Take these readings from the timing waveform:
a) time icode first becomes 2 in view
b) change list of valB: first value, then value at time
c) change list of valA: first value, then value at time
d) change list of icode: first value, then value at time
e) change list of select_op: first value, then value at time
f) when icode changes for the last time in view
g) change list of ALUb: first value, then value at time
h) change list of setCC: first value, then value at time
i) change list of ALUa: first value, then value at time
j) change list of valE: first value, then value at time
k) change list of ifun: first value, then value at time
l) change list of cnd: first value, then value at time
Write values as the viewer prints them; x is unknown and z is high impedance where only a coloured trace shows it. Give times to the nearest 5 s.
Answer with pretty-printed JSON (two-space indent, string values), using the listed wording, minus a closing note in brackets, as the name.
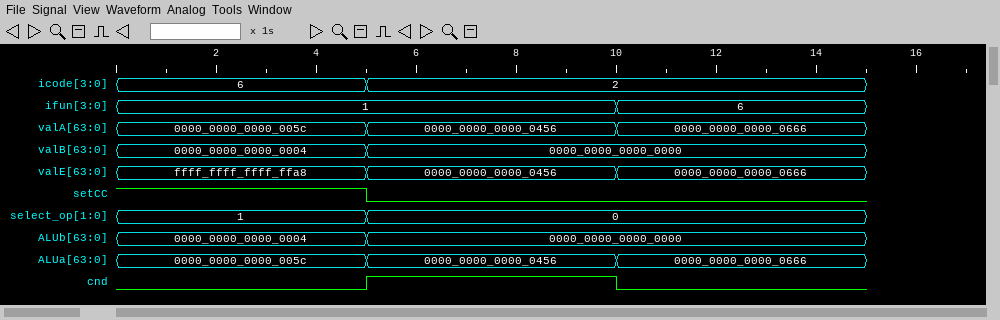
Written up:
{
  "time icode first becomes 2 in view": "5 s",
  "change list of valB: first value, then value at time": "0000_0000_0000_0004, 0000_0000_0000_0000 at 5 s",
  "change list of valA: first value, then value at time": "0000_0000_0000_005c, 0000_0000_0000_0456 at 5 s, 0000_0000_0000_0666 at 10 s",
  "change list of icode: first value, then value at time": "6, 2 at 5 s",
  "change list of select_op: first value, then value at time": "1, 0 at 5 s",
  "when icode changes for the last time in view": "5 s",
  "change list of ALUb: first value, then value at time": "0000_0000_0000_0004, 0000_0000_0000_0000 at 5 s",
  "change list of setCC: first value, then value at time": "1, 0 at 5 s",
  "change list of ALUa: first value, then value at time": "0000_0000_0000_005c, 0000_0000_0000_0456 at 5 s, 0000_0000_0000_0666 at 10 s",
  "change list of valE: first value, then value at time": "ffff_ffff_ffff_ffa8, 0000_0000_0000_0456 at 5 s, 0000_0000_0000_0666 at 10 s",
  "change list of ifun: first value, then value at time": "1, 6 at 10 s",
  "change list of cnd: first value, then value at time": "0, 1 at 5 s, 0 at 10 s"
}
